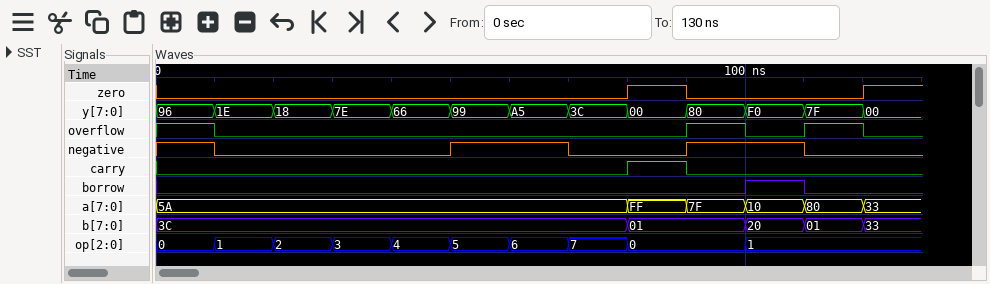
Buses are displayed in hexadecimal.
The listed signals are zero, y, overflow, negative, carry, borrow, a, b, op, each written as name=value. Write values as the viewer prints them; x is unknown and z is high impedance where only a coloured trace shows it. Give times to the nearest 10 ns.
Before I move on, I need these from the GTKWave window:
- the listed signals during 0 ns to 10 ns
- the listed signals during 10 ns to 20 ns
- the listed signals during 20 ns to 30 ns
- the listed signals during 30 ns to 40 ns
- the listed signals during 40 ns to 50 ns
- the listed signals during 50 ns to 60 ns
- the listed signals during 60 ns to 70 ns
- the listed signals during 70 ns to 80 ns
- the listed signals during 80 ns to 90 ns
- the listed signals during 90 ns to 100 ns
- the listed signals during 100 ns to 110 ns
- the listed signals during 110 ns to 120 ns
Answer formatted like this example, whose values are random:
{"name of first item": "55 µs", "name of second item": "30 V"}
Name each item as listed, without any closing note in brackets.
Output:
{"the listed signals during 0 ns to 10 ns": "zero=0, y=96, overflow=1, negative=1, carry=0, borrow=0, a=5A, b=3C, op=0", "the listed signals during 10 ns to 20 ns": "zero=0, y=1E, overflow=0, negative=0, carry=0, borrow=0, a=5A, b=3C, op=1", "the listed signals during 20 ns to 30 ns": "zero=0, y=18, overflow=0, negative=0, carry=0, borrow=0, a=5A, b=3C, op=2", "the listed signals during 30 ns to 40 ns": "zero=0, y=7E, overflow=0, negative=0, carry=0, borrow=0, a=5A, b=3C, op=3", "the listed signals during 40 ns to 50 ns": "zero=0, y=66, overflow=0, negative=0, carry=0, borrow=0, a=5A, b=3C, op=4", "the listed signals during 50 ns to 60 ns": "zero=0, y=99, overflow=0, negative=1, carry=0, borrow=0, a=5A, b=3C, op=5", "the listed signals during 60 ns to 70 ns": "zero=0, y=A5, overflow=0, negative=1, carry=0, borrow=0, a=5A, b=3C, op=6", "the listed signals during 70 ns to 80 ns": "zero=0, y=3C, overflow=0, negative=0, carry=0, borrow=0, a=5A, b=3C, op=7", "the listed signals during 80 ns to 90 ns": "zero=1, y=00, overflow=0, negative=0, carry=1, borrow=0, a=FF, b=01, op=0", "the listed signals during 90 ns to 100 ns": "zero=0, y=80, overflow=1, negative=1, carry=0, borrow=0, a=7F, b=01, op=0", "the listed signals during 100 ns to 110 ns": "zero=0, y=F0, overflow=0, negative=1, carry=0, borrow=1, a=10, b=20, op=1", "the listed signals during 110 ns to 120 ns": "zero=0, y=7F, overflow=1, negative=0, carry=0, borrow=0, a=80, b=01, op=1"}
